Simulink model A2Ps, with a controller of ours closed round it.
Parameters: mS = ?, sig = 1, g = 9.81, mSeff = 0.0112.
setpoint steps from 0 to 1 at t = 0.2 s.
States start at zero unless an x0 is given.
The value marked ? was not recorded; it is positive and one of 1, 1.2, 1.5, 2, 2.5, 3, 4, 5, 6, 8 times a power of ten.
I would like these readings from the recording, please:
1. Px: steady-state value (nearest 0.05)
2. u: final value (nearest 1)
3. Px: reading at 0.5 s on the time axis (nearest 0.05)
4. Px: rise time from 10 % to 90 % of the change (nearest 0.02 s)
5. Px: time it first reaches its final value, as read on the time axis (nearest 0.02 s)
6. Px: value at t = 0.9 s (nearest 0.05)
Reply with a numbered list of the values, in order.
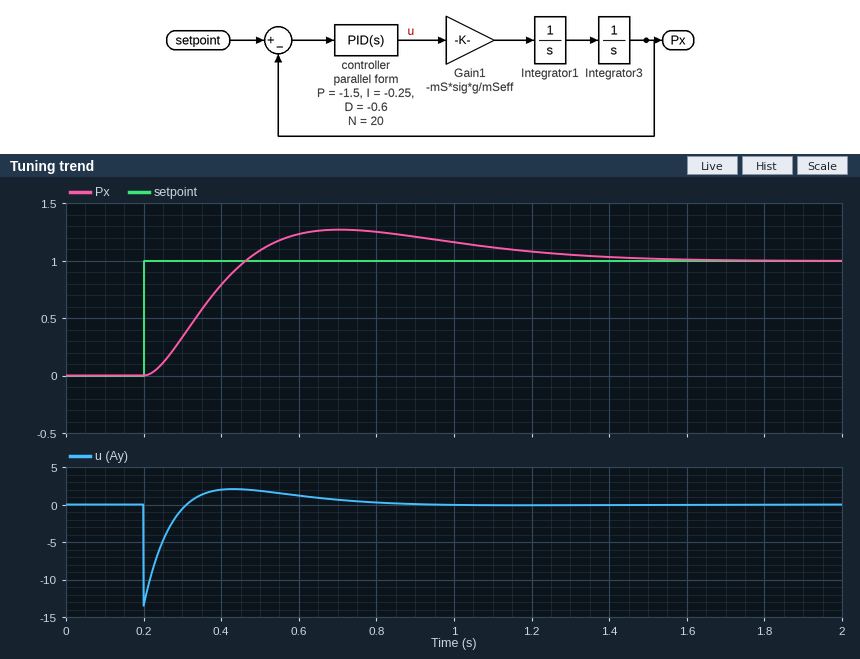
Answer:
1. 1.00
2. 0
3. 1.10
4. 0.18 s
5. 0.46 s
6. 1.20
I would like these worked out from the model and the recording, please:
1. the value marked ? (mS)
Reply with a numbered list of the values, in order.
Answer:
1. 0.01
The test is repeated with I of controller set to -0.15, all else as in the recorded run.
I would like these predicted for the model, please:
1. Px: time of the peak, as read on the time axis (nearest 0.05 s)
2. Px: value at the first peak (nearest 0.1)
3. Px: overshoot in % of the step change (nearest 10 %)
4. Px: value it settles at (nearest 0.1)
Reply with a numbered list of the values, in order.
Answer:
1. 0.70 s
2. 1.3
3. 30 %
4. 1.0
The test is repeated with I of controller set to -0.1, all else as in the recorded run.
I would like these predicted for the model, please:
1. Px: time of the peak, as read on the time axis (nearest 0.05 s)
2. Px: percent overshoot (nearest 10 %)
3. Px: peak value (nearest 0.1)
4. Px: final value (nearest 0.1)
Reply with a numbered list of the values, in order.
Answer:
1. 0.70 s
2. 30 %
3. 1.3
4. 1.0
